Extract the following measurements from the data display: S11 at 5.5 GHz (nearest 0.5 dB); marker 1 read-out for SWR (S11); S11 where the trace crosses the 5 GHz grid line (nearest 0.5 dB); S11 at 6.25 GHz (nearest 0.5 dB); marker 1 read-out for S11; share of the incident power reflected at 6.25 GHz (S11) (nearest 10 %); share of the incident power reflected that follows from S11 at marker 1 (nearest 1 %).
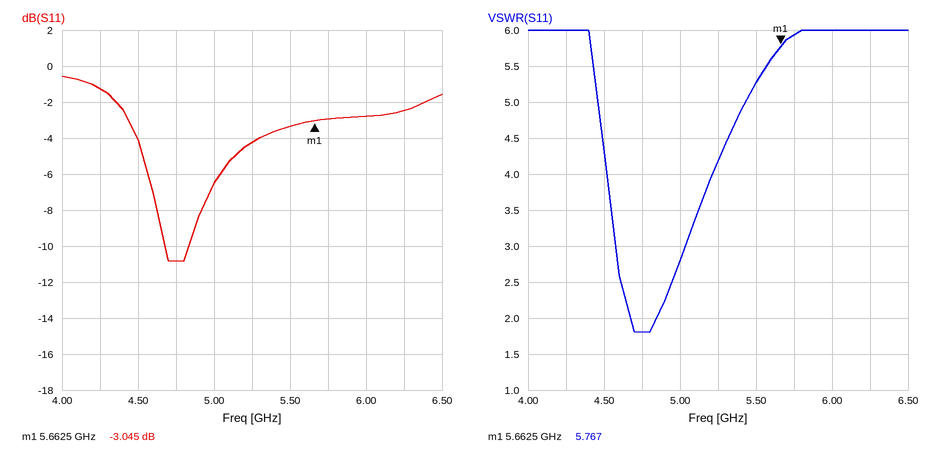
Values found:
-3.5 dB
5.767
-6.5 dB
-2.5 dB
-3.045 dB
60 %
50 %
